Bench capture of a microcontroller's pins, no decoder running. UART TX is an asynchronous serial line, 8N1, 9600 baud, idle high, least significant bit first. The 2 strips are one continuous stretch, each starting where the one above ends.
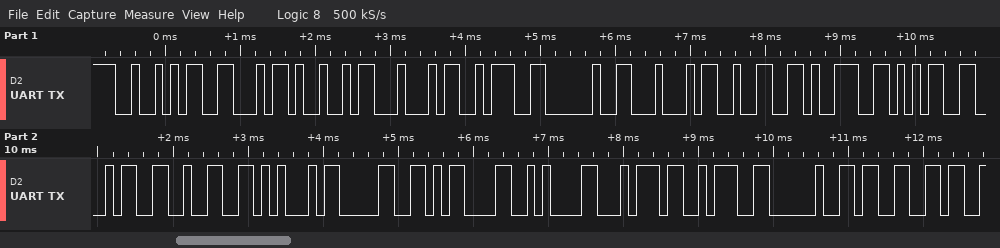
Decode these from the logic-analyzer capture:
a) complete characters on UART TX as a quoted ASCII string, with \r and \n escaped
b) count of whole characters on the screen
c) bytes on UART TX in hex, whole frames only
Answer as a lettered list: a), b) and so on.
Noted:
a) "RFID: D29542E0\r\nt: 3"
b) 20
c) 0x52 0x46 0x49 0x44 0x3A 0x20 0x44 0x32 0x39 0x35 0x34 0x32 0x45 0x30 0x0D 0x0A 0x74 0x3A 0x20 0x33
